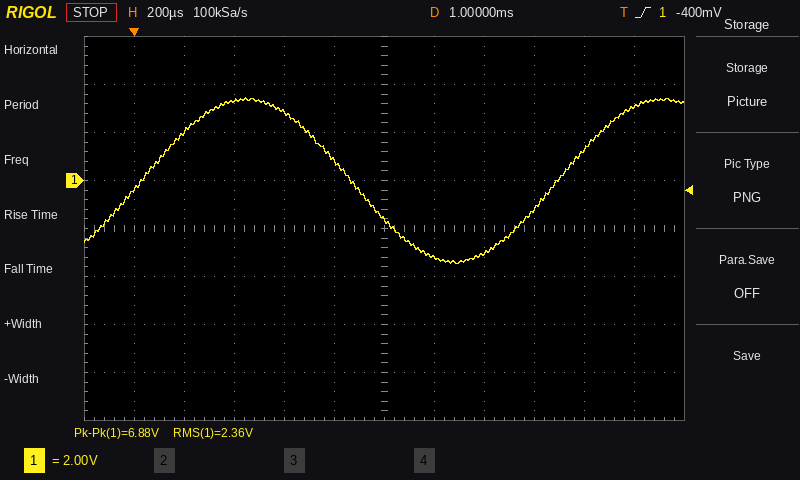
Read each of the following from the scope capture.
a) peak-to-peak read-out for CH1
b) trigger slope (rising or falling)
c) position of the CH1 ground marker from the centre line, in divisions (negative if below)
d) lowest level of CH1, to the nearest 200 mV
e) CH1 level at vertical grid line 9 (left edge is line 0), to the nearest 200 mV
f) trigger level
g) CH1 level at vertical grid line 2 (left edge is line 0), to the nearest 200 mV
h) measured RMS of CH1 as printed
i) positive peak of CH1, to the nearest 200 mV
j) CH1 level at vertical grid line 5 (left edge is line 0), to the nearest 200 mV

6.88 V
rising
+1.0 div
-3.4 V
-1.2 V
-400 mV
2.0 V
2.36 V
3.4 V
800 mV
